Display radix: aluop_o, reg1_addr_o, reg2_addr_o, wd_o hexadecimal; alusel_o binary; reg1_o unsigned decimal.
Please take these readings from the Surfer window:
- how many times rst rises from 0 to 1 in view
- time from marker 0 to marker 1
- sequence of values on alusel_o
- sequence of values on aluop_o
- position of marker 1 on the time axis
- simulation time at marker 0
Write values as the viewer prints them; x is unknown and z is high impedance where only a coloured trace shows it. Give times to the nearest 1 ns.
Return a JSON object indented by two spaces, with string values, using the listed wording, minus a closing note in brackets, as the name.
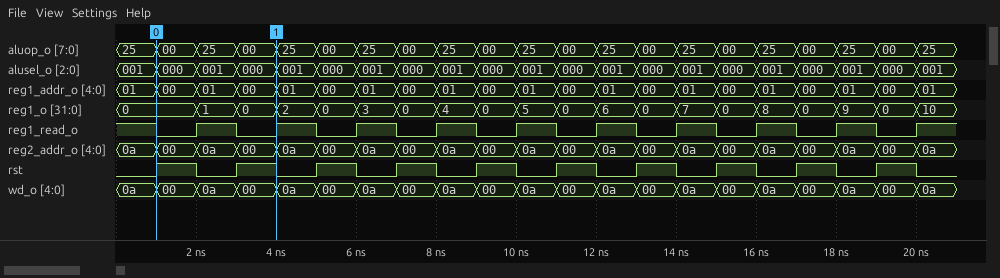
{
  "how many times rst rises from 0 to 1 in view": "10",
  "time from marker 0 to marker 1": "3 ns",
  "sequence of values on alusel_o": "001, 000, 001, 000, 001, 000, 001, 000, 001, 000, 001, 000, 001, 000, 001, 000, 001, 000, 001, 000, 001",
  "sequence of values on aluop_o": "25, 00, 25, 00, 25, 00, 25, 00, 25, 00, 25, 00, 25, 00, 25, 00, 25, 00, 25, 00, 25",
  "position of marker 1 on the time axis": "4 ns",
  "simulation time at marker 0": "1 ns"
}
